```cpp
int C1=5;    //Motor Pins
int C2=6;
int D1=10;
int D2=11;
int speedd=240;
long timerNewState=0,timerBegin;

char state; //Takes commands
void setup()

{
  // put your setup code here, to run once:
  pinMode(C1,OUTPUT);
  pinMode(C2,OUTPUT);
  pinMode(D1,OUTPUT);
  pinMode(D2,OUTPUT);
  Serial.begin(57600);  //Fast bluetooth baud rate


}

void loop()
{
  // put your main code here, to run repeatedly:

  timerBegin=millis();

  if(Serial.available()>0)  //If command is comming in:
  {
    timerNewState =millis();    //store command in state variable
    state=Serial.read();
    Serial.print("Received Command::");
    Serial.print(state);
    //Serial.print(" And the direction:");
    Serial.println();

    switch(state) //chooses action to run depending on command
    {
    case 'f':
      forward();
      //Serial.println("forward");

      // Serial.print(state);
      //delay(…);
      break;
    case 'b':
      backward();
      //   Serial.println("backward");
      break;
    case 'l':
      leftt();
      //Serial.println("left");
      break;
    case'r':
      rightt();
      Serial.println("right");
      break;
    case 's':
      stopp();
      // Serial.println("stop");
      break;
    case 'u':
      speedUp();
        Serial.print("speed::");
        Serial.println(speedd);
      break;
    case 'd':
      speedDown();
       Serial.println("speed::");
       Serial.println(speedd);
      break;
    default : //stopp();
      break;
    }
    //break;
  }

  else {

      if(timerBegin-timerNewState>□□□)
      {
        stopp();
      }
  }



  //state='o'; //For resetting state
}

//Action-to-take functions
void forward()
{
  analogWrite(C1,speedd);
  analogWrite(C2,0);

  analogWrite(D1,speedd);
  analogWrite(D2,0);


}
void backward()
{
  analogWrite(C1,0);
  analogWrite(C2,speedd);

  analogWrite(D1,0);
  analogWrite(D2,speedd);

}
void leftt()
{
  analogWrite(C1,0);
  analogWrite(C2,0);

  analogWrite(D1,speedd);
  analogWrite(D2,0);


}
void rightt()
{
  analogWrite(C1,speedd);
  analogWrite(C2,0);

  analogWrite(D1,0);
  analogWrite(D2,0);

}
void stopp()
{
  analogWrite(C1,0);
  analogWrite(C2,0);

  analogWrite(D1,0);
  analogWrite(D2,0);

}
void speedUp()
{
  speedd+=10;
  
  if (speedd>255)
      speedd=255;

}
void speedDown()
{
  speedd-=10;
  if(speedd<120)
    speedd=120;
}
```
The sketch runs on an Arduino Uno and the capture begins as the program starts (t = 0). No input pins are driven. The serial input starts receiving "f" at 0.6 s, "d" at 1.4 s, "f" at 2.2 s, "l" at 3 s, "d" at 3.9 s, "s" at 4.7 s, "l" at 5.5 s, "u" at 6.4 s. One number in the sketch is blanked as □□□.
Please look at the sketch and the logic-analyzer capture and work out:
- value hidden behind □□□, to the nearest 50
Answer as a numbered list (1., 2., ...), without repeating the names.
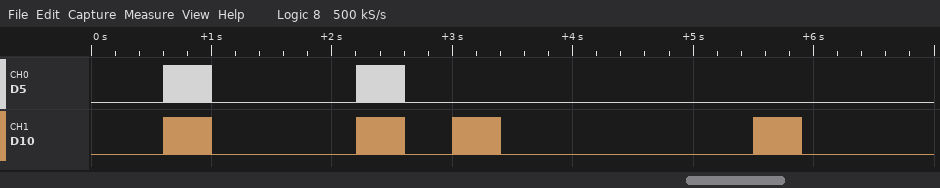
1. 400
